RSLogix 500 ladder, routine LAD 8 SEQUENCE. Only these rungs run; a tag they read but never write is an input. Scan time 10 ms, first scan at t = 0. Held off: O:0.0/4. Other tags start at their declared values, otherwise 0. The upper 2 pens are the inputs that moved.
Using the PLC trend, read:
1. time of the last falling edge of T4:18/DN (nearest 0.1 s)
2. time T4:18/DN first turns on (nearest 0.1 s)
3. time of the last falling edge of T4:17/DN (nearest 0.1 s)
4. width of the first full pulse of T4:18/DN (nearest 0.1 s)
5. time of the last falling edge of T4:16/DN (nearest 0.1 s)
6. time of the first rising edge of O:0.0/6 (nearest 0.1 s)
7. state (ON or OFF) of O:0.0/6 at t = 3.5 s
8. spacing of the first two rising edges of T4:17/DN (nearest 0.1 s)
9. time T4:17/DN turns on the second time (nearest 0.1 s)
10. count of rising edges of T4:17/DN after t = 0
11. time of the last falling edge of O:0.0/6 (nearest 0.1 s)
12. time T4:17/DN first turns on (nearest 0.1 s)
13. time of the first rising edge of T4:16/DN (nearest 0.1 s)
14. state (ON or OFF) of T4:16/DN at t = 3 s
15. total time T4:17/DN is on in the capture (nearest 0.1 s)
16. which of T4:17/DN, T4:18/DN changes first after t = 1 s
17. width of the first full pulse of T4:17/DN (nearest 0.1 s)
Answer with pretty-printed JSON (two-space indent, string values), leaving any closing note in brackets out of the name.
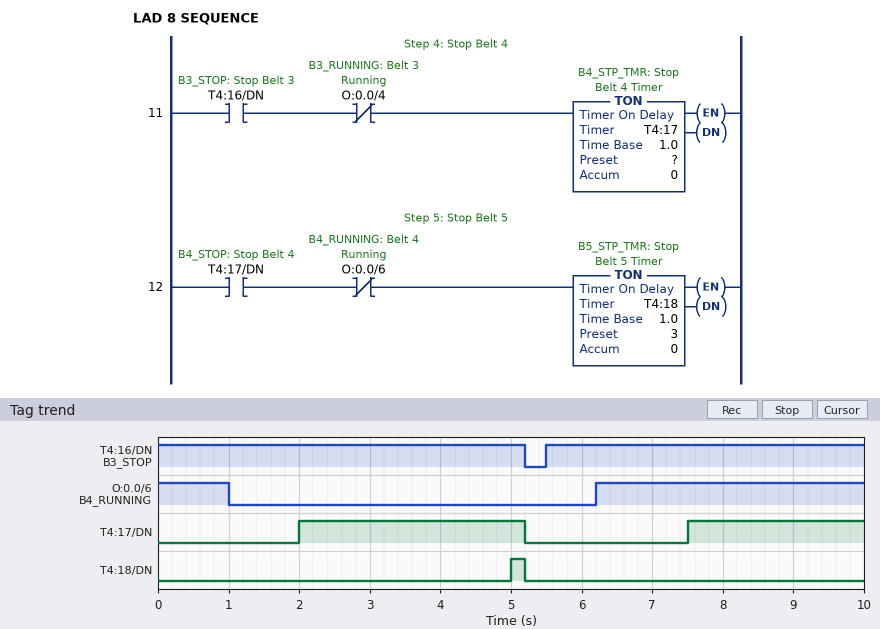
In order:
{
  "time of the last falling edge of T4:18/DN": "5.2 s",
  "time T4:18/DN first turns on": "5.0 s",
  "time of the last falling edge of T4:17/DN": "5.2 s",
  "width of the first full pulse of T4:18/DN": "0.2 s",
  "time of the last falling edge of T4:16/DN": "5.2 s",
  "time of the first rising edge of O:0.0/6": "6.2 s",
  "state (ON or OFF) of O:0.0/6 at t = 3.5 s": "OFF",
  "spacing of the first two rising edges of T4:17/DN": "5.5 s",
  "time T4:17/DN turns on the second time": "7.5 s",
  "count of rising edges of T4:17/DN after t = 0": "2",
  "time of the last falling edge of O:0.0/6": "1.0 s",
  "time T4:17/DN first turns on": "2.0 s",
  "time of the first rising edge of T4:16/DN": "5.5 s",
  "state (ON or OFF) of T4:16/DN at t = 3 s": "ON",
  "total time T4:17/DN is on in the capture": "5.7 s",
  "which of T4:17/DN, T4:18/DN changes first after t = 1 s": "T4:17/DN",
  "width of the first full pulse of T4:17/DN": "3.2 s"
}
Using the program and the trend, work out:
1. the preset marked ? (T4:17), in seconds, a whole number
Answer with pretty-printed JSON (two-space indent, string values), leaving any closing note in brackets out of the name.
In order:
{
  "the preset marked ? (T4:17), in seconds, a whole number": "2 s"
}
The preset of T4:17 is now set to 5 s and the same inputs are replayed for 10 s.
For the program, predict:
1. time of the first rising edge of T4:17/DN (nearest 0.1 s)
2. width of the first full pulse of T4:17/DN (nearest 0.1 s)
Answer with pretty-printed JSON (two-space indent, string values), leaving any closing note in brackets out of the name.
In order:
{
  "time of the first rising edge of T4:17/DN": "5.0 s",
  "width of the first full pulse of T4:17/DN": "0.2 s"
}
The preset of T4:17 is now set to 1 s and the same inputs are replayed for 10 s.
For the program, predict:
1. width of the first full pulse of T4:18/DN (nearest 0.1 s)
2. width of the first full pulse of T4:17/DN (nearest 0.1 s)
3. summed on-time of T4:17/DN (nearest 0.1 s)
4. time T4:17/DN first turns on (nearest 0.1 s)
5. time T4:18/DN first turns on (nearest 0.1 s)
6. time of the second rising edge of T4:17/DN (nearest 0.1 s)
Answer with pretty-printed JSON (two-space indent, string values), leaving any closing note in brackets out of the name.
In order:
{
  "width of the first full pulse of T4:18/DN": "1.2 s",
  "width of the first full pulse of T4:17/DN": "4.2 s",
  "summed on-time of T4:17/DN": "7.7 s",
  "time T4:17/DN first turns on": "1.0 s",
  "time T4:18/DN first turns on": "4.0 s",
  "time of the second rising edge of T4:17/DN": "6.5 s"
}
